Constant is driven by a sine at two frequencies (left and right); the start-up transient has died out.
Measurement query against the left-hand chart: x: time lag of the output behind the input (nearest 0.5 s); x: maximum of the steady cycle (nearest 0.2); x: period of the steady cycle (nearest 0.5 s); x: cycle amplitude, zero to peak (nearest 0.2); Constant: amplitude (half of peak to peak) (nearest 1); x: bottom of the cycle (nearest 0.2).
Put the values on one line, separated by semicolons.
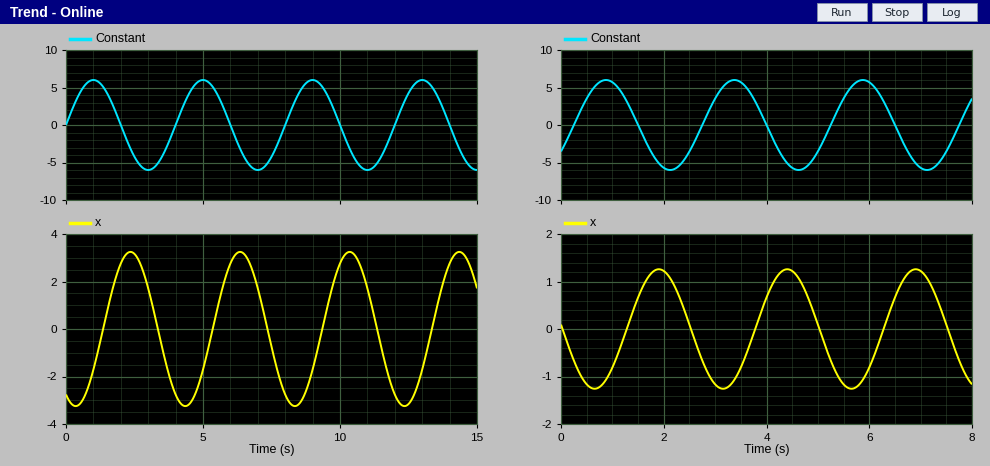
1.5 s; 3.2; 4.0 s; 3.2; 6; -3.2
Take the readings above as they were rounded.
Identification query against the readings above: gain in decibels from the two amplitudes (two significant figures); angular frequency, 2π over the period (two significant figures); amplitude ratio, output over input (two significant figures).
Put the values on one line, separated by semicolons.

-5.5 dB; 1.6 rad/s; 0.53
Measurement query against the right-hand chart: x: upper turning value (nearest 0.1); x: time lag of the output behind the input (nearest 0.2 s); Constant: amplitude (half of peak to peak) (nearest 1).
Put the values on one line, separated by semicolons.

1.3; 1.0 s; 6
